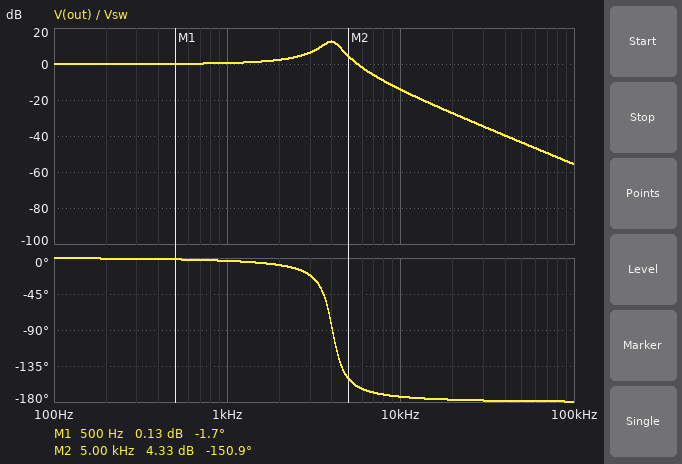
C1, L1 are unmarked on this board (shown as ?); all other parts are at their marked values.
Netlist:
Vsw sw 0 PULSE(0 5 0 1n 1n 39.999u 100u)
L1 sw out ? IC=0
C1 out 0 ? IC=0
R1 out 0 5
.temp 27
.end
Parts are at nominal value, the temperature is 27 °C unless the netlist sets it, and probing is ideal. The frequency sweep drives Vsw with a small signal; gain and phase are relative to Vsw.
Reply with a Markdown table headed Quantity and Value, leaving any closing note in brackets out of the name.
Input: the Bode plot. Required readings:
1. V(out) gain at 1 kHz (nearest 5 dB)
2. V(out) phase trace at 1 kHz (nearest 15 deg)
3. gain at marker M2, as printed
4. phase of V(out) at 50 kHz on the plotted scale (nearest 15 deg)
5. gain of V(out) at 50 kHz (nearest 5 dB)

| Quantity | Value |
|---|---|
| V(out) gain at 1 kHz | 0 dB |
| V(out) phase trace at 1 kHz | 0 deg |
| gain at marker M2, as printed | 4.33 dB |
| phase of V(out) at 50 kHz on the plotted scale | -180 deg |
| gain of V(out) at 50 kHz | -45 dB |
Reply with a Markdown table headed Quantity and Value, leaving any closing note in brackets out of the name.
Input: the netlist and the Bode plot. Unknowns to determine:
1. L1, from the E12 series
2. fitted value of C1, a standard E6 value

| Quantity | Value |
|---|---|
| L1, from the E12 series | 47 µH |
| fitted value of C1, a standard E6 value | 33 µF |
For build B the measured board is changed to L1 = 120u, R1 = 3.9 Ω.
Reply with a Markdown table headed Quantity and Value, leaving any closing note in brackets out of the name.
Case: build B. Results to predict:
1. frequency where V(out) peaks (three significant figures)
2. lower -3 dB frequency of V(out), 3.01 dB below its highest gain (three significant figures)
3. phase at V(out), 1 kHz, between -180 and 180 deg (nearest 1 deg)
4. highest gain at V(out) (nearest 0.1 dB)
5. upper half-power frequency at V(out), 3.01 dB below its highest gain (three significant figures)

| Quantity | Value |
|---|---|
| frequency where V(out) peaks | 2.37 kHz |
| lower -3 dB frequency of V(out), 3.01 dB below its highest gain | 1.61 kHz |
| phase at V(out), 1 kHz, between -180 and 180 deg | -13 deg |
| highest gain at V(out) | 6.5 dB |
| upper half-power frequency at V(out), 3.01 dB below its highest gain | 2.94 kHz |
